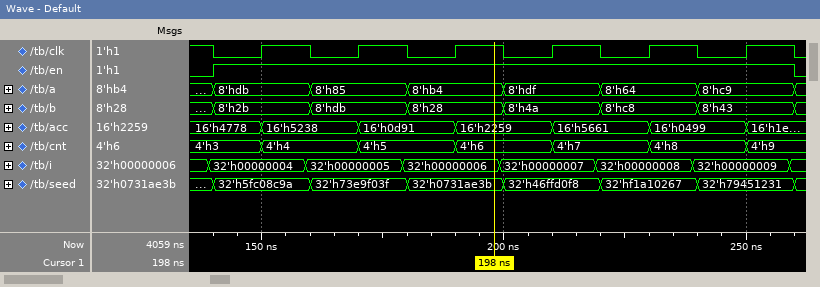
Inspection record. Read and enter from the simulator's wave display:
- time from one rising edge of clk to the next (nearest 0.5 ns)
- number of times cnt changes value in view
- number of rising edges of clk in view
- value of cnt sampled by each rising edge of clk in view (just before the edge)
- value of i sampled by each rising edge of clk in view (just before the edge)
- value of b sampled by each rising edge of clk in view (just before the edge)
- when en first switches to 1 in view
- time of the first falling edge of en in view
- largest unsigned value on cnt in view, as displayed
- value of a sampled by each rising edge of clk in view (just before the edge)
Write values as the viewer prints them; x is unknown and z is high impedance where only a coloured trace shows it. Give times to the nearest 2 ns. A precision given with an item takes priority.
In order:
20 ns
6
6
4'h3, 4'h4, 4'h5, 4'h6, 4'h7, 4'h8
32'h00000004, 32'h00000005, 32'h00000006, 32'h00000007, 32'h00000008, 32'h00000009
8'h2b, 8'hdb, 8'h28, 8'h4a, 8'hc8, 8'h43
140 ns
260 ns
4'h9
8'hdb, 8'h85, 8'hb4, 8'hdf, 8'h64, 8'hc9
